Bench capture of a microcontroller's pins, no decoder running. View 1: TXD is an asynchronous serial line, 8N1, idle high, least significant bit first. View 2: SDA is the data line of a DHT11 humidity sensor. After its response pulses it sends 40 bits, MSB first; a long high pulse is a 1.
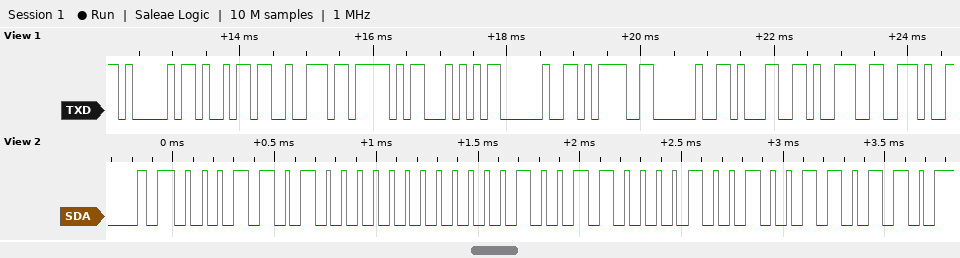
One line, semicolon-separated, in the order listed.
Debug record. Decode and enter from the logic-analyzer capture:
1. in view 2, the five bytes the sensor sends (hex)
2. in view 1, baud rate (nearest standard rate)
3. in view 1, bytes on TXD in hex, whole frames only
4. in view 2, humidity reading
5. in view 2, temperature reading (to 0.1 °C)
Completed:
1A 00 13 09 36; 9600 baud; 41 69 72 5F 54 20 3D 20 31 39 2E; 26 %; 19.9 °C
